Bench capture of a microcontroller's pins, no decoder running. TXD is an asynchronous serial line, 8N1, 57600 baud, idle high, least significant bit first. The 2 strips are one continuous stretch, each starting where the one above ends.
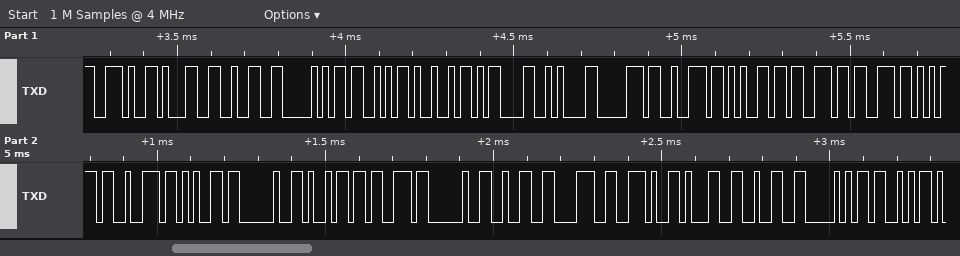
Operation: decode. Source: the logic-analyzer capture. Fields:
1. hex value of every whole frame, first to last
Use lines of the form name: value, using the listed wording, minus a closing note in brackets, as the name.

hex value of every whole frame, first to last: 2E 31 32 50 53 49 0D 0A 70 72 65 73 73 75 72 65 20 69 73 20 32 38 2E 31 32 50 53
